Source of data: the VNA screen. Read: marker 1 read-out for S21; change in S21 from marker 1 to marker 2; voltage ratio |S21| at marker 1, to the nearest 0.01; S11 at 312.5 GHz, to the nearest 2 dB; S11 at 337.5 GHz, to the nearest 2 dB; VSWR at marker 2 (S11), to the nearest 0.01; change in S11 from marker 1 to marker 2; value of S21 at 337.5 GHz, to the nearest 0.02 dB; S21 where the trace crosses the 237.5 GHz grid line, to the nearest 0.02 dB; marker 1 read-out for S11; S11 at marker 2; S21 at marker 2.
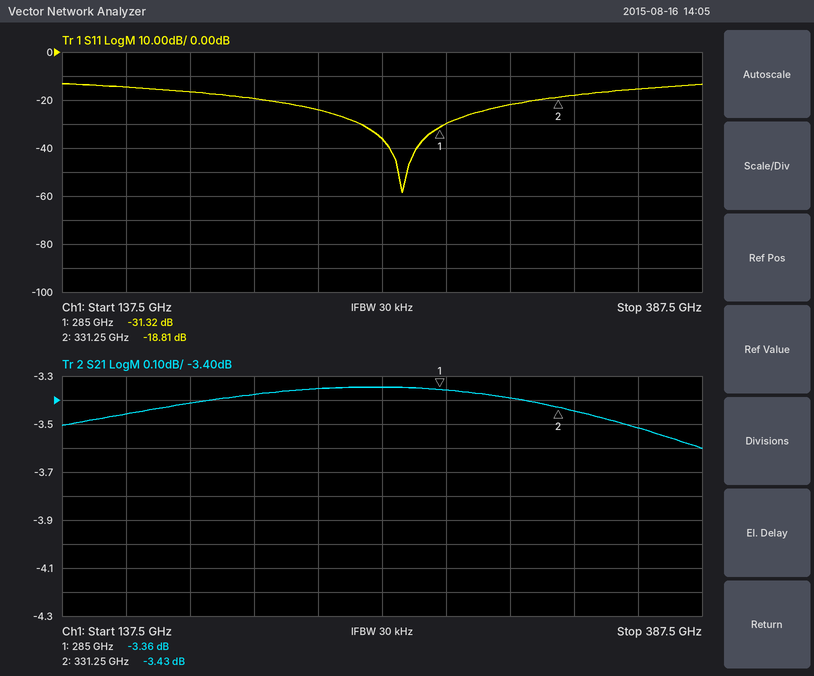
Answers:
-3.36 dB
-0.07 dB
0.68
-22 dB
-18 dB
1.26
12.51 dB
-3.44 dB
-3.36 dB
-31.32 dB
-18.81 dB
-3.43 dB
